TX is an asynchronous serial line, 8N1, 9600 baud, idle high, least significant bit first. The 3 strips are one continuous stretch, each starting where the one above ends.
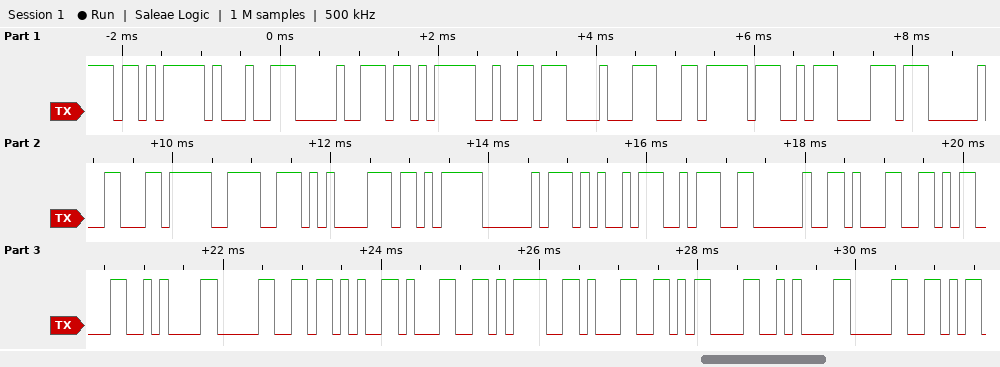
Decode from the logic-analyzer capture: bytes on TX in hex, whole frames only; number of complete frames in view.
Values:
0xEB 0x91 0x90 0xEB 0xB2 0x88 0xEC 0xA7 0xB8 0x20 0xEC 0x9E 0x85 0xEB 0xA0 0xA5 0x3A 0x20 0x31 0x0D 0x0A 0x30 0x2B 0x31 0x3D 0x31 0x0D 0x0A 0x30
29
